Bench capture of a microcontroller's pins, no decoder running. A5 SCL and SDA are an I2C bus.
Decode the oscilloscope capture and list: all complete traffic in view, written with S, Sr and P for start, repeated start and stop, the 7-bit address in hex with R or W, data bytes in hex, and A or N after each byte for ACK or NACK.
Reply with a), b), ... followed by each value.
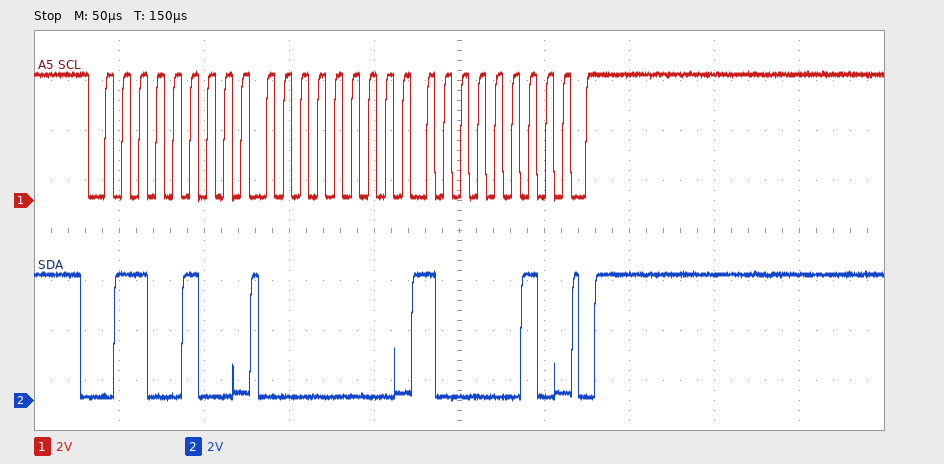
a) S 32W A 00 A 82 A P
